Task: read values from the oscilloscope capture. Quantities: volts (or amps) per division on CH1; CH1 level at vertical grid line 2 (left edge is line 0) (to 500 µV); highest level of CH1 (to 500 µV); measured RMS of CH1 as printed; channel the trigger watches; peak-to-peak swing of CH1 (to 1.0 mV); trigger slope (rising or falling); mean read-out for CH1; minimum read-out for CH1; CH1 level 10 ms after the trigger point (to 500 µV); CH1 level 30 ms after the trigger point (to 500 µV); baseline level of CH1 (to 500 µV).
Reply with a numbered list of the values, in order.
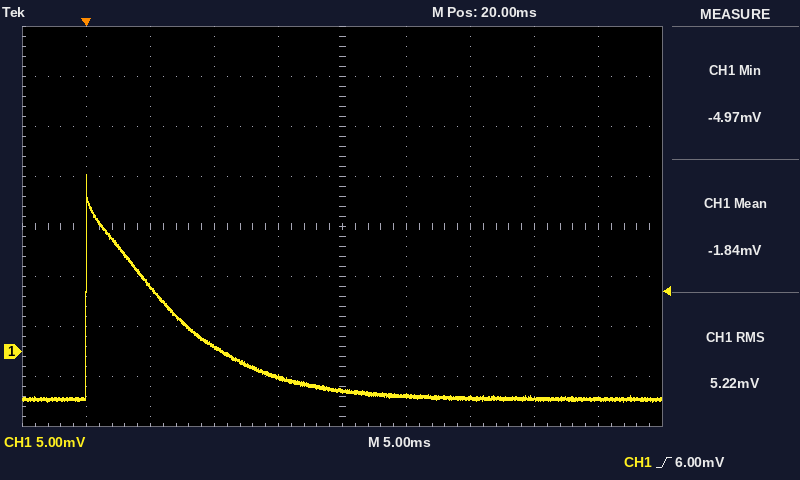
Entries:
1. 5 mV
2. 6.5 mV
3. 17.5 mV
4. 5.22 mV
5. CH1
6. 23.0 mV
7. rising
8. -1.84 mV
9. -4.97 mV
10. 500 µV
11. -4.5 mV
12. -4.5 mV
